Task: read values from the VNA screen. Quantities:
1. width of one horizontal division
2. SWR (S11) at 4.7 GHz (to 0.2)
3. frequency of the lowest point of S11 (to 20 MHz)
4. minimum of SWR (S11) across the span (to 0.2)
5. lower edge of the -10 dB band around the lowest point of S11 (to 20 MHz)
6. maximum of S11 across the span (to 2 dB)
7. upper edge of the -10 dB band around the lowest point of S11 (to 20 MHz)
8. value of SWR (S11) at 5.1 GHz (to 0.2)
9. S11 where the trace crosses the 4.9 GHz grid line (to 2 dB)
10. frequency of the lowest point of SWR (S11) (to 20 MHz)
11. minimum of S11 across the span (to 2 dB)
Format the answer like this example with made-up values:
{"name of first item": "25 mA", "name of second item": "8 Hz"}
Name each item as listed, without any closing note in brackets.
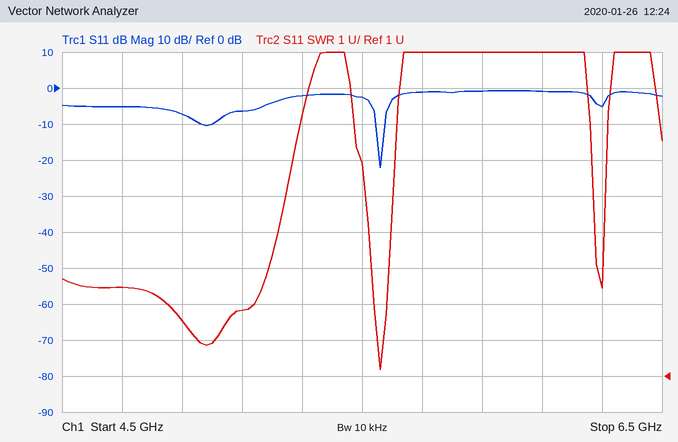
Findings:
{"width of one horizontal division": "200 MHz", "SWR (S11) at 4.7 GHz": "3.4", "frequency of the lowest point of S11": "5.56 GHz", "minimum of SWR (S11) across the span": "1.2", "lower edge of the -10 dB band around the lowest point of S11": "5.54 GHz", "maximum of S11 across the span": "0 dB", "upper edge of the -10 dB band around the lowest point of S11": "5.58 GHz", "value of SWR (S11) at 5.1 GHz": "2.8", "S11 where the trace crosses the 4.9 GHz grid line": "-8 dB", "frequency of the lowest point of SWR (S11)": "5.56 GHz", "minimum of S11 across the span": "-22 dB"}
